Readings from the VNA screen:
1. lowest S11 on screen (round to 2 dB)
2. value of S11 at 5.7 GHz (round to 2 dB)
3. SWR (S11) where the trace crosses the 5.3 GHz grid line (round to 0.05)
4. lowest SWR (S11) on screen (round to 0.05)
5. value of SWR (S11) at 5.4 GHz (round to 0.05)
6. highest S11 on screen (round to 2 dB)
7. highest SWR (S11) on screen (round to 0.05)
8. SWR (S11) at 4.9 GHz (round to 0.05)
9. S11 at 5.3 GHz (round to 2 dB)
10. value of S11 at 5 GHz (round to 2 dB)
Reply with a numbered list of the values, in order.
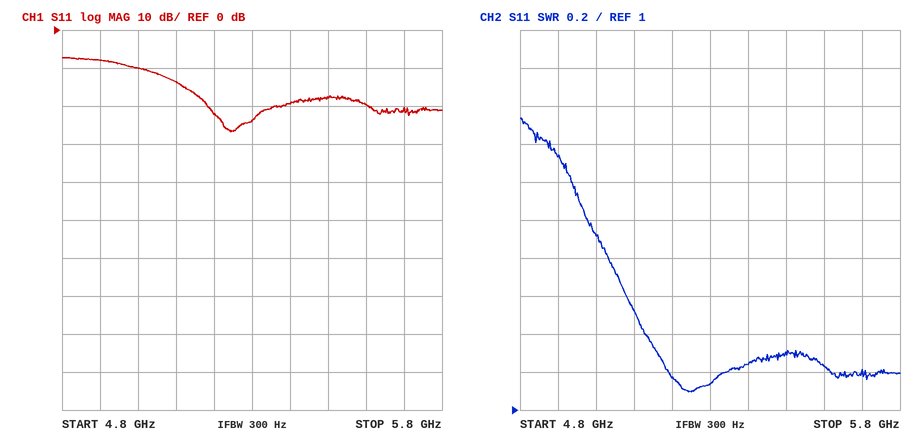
1. -26 dB
2. -20 dB
3. 1.15
4. 1.10
5. 1.25
6. -8 dB
7. 2.55
8. 2.35
9. -24 dB
10. -10 dB
